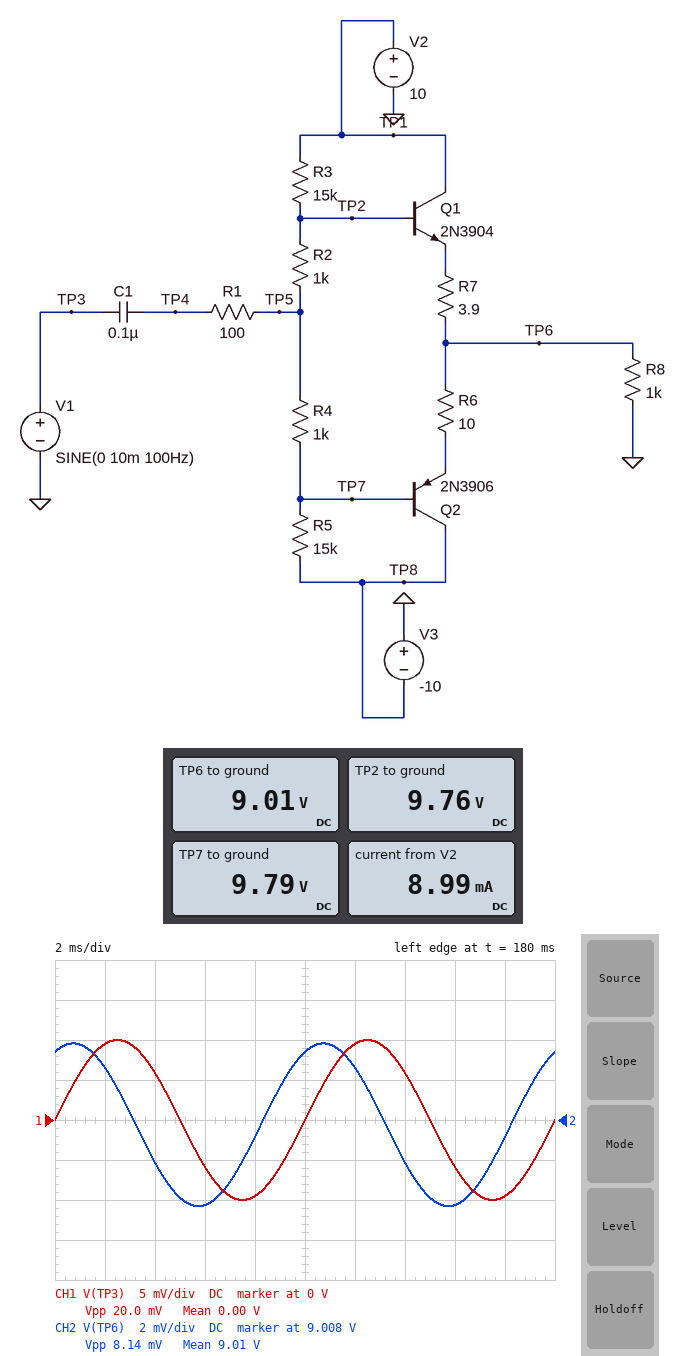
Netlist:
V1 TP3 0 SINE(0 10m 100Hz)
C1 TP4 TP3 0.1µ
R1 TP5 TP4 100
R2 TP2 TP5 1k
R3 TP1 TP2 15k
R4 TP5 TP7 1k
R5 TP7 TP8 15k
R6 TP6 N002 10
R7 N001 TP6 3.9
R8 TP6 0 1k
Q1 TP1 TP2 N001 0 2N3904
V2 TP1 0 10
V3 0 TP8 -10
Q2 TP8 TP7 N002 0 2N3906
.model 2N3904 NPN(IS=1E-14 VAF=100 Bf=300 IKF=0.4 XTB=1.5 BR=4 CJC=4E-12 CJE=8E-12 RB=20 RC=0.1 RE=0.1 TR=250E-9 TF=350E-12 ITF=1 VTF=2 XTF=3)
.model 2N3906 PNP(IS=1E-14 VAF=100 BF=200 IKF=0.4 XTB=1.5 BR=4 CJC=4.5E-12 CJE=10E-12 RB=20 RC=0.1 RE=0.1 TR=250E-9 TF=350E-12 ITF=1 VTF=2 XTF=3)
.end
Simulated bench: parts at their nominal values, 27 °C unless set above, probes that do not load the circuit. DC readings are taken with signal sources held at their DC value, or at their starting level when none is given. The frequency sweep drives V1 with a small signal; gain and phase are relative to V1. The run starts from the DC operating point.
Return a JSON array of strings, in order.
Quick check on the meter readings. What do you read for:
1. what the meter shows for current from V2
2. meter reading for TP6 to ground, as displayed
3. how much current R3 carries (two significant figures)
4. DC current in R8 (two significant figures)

["8.99 mA", "9.01 V", "16 µA", "9.0 mA"]
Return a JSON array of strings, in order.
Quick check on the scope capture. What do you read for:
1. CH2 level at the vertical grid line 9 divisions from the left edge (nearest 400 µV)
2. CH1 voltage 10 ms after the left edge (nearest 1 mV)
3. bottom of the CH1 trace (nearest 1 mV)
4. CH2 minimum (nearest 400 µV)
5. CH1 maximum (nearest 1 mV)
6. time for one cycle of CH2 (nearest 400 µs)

["9.0072 V", "0 V", "-10 mV", "9.0036 V", "10 mV", "10.0 ms"]
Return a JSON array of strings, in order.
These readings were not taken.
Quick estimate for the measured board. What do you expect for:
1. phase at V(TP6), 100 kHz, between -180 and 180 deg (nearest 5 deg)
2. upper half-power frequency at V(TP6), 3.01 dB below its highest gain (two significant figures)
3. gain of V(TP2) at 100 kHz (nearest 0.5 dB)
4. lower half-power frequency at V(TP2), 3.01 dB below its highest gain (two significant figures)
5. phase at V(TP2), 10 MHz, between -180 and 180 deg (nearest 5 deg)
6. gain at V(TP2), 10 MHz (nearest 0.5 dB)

["0 deg", "35 MHz", "-0.5 dB", "200 Hz", "-15 deg", "-1.0 dB"]
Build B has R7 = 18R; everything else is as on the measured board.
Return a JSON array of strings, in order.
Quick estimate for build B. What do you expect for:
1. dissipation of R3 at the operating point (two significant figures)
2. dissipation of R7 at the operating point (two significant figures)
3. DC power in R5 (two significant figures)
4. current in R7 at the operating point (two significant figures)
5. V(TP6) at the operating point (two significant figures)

["3.8 µW", "1.4 mW", "3.0 µW", "8.9 mA", "8.9 V"]
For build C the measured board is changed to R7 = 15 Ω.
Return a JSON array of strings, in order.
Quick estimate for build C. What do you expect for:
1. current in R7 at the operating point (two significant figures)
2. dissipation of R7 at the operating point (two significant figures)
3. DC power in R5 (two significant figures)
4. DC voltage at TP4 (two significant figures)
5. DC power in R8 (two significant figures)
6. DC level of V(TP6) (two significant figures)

["8.9 mA", "1.2 mW", "3.0 µW", "9.8 V", "79 mW", "8.9 V"]
